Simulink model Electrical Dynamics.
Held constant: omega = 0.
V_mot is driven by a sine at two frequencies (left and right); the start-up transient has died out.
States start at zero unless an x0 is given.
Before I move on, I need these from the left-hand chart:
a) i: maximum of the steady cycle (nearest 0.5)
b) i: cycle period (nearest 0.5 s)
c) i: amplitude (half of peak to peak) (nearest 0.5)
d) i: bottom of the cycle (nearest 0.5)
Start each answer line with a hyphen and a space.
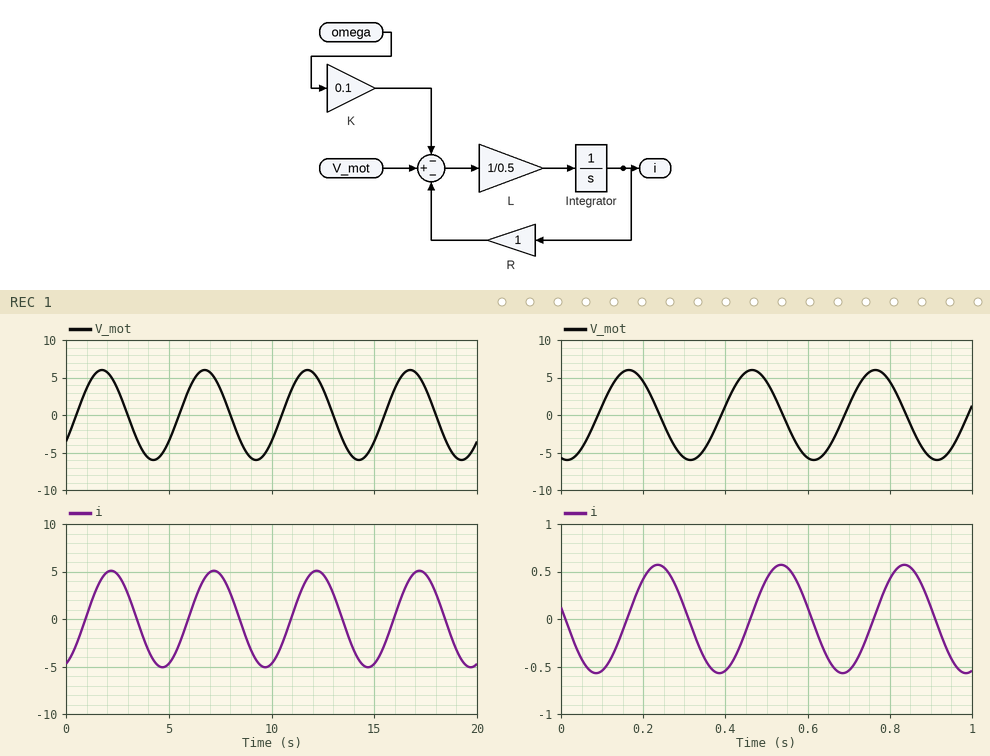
- 5.0
- 5.0 s
- 5.0
- -5.0
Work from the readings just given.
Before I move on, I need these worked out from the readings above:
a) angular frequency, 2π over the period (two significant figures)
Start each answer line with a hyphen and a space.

- 1.3 rad/s
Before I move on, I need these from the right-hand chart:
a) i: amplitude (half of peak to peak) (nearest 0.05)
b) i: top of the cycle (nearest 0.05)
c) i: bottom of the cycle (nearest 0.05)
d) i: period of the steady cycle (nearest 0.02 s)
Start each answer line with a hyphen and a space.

- 0.55
- 0.55
- -0.55
- 0.30 s
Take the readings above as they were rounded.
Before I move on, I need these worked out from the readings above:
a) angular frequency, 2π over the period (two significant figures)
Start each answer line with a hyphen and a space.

- 21 rad/s
